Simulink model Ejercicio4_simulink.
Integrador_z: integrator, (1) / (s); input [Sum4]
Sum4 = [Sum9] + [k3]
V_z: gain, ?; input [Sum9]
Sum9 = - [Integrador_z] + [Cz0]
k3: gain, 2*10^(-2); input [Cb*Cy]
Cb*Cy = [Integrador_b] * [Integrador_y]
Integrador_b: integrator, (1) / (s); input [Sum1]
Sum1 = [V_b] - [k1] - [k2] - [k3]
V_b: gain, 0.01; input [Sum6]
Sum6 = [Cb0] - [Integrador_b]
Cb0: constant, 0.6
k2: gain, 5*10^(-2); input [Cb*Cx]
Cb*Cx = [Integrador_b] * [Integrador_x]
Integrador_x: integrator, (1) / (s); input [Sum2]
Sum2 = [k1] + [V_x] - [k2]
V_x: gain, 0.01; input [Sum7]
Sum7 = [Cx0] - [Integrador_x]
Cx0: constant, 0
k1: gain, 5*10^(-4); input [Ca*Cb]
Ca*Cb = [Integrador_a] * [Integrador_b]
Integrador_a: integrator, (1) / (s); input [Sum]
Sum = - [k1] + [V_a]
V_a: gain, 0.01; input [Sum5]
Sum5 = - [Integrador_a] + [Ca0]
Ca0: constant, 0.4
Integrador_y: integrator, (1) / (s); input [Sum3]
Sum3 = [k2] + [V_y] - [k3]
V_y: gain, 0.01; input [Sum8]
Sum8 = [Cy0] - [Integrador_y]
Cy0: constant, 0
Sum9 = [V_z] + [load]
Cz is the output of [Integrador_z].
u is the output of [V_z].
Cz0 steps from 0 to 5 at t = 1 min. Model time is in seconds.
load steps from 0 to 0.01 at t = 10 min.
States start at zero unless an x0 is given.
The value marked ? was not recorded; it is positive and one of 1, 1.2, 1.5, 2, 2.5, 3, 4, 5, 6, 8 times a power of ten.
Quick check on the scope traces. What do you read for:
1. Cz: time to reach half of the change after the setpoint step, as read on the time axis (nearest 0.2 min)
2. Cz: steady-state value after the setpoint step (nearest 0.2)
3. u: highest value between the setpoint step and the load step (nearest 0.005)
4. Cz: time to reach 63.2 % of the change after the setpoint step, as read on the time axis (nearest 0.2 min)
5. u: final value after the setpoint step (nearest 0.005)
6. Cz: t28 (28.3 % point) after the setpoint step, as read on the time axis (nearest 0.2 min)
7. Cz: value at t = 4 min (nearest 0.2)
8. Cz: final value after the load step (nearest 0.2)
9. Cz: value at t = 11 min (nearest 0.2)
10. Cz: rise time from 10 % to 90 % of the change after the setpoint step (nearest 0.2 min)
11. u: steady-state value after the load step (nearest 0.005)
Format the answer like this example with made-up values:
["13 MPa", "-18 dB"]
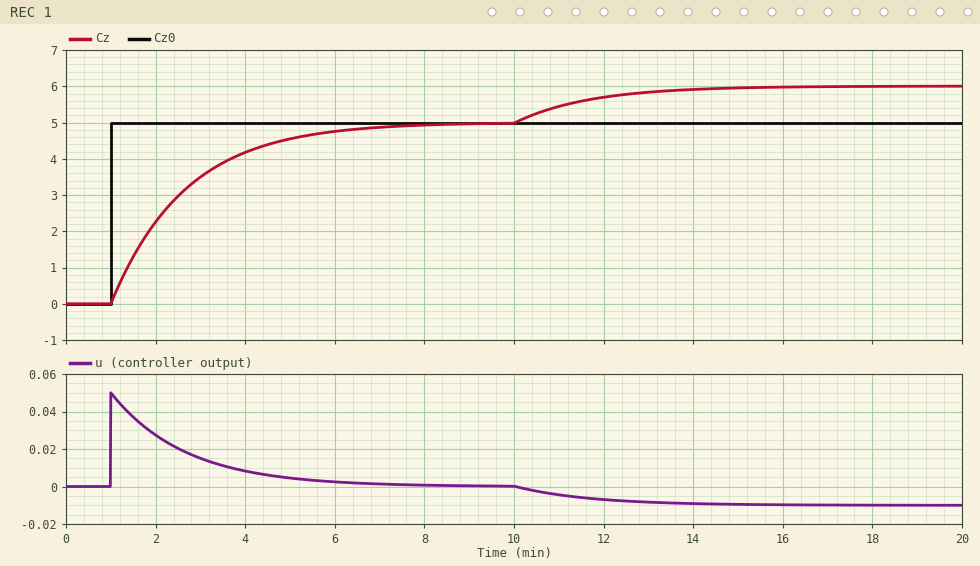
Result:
["2.2 min", "5.0", "0.050", "2.6 min", "0.000", "1.6 min", "4.2", "6.0", "5.4", "3.6 min", "-0.010"]
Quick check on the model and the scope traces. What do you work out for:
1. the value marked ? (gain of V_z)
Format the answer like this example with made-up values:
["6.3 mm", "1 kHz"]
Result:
["0.01"]
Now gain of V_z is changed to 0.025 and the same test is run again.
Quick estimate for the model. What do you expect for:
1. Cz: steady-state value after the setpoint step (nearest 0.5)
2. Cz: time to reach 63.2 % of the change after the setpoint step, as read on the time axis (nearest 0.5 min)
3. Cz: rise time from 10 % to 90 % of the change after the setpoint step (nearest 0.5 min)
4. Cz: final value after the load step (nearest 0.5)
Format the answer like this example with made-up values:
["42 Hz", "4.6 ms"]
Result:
["5.0", "1.5 min", "1.5 min", "5.5"]
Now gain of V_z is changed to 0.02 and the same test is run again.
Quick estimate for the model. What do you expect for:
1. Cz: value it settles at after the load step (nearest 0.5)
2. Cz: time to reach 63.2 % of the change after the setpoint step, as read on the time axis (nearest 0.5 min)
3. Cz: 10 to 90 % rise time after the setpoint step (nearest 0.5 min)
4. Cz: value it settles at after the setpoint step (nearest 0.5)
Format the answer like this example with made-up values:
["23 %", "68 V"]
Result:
["5.5", "2.0 min", "2.0 min", "5.0"]
